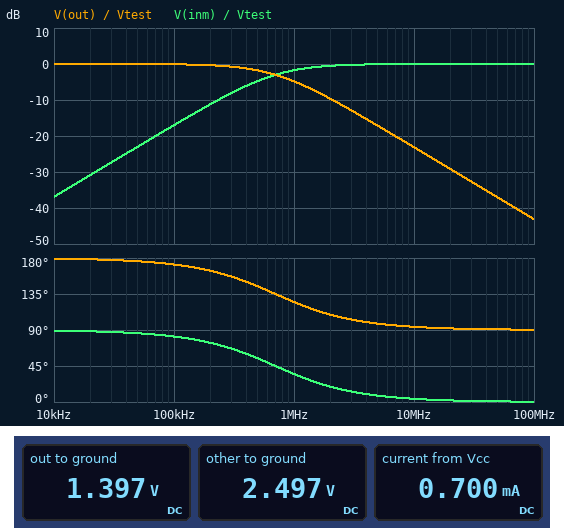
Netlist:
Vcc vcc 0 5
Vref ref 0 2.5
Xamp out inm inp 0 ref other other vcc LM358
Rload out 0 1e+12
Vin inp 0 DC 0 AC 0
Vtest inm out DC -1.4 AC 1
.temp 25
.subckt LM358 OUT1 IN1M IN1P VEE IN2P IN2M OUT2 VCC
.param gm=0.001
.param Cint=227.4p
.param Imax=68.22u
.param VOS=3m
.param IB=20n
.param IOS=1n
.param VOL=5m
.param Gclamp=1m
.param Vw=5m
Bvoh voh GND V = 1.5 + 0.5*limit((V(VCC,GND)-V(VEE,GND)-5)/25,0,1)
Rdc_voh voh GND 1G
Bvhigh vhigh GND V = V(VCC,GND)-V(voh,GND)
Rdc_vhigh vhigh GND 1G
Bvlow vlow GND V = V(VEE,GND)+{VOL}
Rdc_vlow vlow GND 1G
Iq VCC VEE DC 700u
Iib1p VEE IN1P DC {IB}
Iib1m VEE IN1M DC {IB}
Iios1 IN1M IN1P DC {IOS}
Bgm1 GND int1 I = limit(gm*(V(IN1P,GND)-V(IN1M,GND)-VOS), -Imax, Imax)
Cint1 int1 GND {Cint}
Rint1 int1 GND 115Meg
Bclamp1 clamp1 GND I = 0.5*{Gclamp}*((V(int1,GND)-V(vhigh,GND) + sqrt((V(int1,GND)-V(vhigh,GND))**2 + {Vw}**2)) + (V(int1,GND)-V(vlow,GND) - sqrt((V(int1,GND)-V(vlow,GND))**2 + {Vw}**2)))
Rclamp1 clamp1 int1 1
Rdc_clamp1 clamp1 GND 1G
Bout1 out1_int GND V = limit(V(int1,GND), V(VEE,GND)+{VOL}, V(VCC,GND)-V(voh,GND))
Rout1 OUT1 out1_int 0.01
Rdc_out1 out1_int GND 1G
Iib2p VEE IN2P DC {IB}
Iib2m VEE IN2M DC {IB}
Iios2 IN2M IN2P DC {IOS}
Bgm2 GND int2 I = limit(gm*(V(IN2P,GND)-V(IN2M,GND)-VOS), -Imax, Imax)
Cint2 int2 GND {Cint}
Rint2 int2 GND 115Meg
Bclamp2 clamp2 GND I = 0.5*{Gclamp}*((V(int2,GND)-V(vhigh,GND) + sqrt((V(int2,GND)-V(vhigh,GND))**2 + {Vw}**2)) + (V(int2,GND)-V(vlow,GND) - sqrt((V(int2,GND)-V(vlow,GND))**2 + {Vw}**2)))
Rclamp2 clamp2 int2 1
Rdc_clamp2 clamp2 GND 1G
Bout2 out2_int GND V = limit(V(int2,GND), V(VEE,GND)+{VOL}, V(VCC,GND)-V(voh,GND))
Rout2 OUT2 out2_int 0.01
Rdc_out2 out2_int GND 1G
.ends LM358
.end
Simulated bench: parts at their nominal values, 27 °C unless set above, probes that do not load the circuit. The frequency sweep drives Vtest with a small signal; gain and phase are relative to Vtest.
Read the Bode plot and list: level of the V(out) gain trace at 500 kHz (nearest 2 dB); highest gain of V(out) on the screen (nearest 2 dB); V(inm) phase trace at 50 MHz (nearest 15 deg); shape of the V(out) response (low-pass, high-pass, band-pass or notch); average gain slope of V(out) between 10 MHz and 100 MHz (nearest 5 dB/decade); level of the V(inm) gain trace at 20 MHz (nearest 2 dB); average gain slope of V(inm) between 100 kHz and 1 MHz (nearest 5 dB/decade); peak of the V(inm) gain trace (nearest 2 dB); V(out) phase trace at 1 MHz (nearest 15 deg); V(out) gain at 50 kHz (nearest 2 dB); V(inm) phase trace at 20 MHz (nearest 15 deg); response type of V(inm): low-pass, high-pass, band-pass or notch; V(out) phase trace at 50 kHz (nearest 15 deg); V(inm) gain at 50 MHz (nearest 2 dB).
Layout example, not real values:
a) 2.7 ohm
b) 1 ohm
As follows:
a) -2 dB
b) 0 dB
c) 0 deg
d) low-pass
e) -20 dB/decade
f) 0 dB
g) 15 dB/decade
h) 0 dB
i) 120 deg
j) 0 dB
k) 0 deg
l) high-pass
m) 180 deg
n) 0 dB
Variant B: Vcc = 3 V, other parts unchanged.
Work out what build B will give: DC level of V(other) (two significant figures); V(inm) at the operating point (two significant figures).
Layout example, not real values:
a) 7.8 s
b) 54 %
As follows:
a) 1.5 V
b) -3.1 mV
